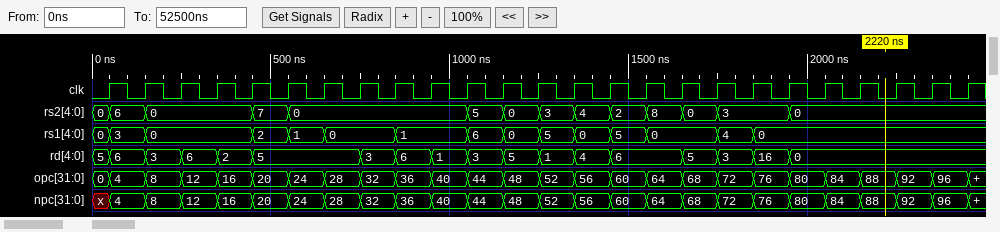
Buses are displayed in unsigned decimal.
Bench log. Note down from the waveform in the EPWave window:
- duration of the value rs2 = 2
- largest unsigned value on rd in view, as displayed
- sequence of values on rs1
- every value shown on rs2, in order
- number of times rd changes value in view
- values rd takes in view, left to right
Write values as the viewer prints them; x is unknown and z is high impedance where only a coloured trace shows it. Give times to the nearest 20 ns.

100 ns
16
0, 3, 0, 2, 1, 0, 1, 6, 0, 5, 0, 5, 0, 4, 0
0, 6, 0, 7, 0, 5, 0, 3, 4, 2, 8, 0, 3, 0
17
5, 6, 3, 6, 2, 5, 3, 6, 1, 3, 5, 1, 4, 6, 5, 3, 16, 0
